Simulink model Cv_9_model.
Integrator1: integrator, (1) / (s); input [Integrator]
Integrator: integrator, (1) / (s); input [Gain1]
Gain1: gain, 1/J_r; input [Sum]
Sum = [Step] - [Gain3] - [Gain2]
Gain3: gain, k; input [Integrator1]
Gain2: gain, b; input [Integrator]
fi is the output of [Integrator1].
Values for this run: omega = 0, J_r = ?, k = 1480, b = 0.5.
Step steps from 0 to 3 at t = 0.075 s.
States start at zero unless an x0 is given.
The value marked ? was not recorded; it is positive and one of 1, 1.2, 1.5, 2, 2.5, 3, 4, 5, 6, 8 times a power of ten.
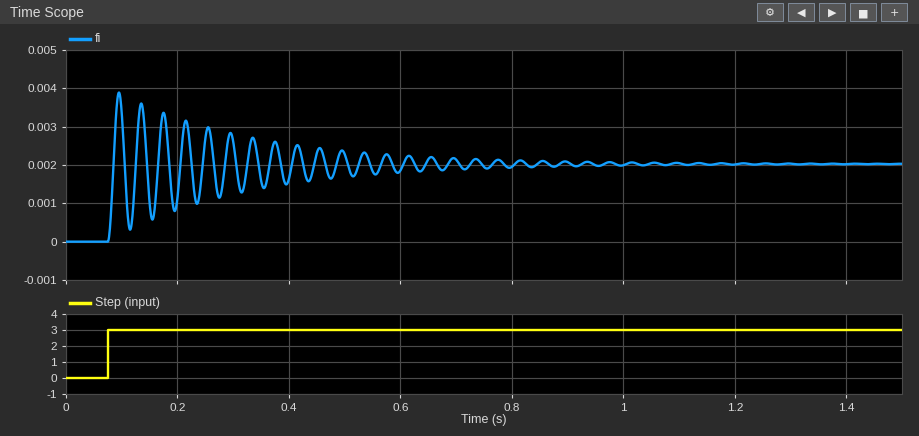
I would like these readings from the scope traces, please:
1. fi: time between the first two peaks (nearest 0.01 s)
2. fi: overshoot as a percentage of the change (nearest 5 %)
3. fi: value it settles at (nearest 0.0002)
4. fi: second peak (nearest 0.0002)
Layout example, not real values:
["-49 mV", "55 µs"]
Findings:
["0.04 s", "90 %", "0.0020", "0.0036"]
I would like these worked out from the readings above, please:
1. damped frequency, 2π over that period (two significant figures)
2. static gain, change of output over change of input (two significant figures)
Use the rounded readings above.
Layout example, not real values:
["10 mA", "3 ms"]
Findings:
["160 rad/s", "0.00067"]
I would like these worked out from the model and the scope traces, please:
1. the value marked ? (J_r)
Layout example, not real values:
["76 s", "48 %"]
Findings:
["0.06"]
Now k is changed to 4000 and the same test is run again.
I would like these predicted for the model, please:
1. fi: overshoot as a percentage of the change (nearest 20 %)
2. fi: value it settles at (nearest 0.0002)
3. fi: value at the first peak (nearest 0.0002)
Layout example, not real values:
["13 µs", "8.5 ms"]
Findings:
["100 %", "0.0008", "0.0014"]
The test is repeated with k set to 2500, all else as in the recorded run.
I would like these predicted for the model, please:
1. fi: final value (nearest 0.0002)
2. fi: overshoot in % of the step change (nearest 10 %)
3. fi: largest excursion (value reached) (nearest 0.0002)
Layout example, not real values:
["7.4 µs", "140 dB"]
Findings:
["0.0012", "90 %", "0.0024"]
